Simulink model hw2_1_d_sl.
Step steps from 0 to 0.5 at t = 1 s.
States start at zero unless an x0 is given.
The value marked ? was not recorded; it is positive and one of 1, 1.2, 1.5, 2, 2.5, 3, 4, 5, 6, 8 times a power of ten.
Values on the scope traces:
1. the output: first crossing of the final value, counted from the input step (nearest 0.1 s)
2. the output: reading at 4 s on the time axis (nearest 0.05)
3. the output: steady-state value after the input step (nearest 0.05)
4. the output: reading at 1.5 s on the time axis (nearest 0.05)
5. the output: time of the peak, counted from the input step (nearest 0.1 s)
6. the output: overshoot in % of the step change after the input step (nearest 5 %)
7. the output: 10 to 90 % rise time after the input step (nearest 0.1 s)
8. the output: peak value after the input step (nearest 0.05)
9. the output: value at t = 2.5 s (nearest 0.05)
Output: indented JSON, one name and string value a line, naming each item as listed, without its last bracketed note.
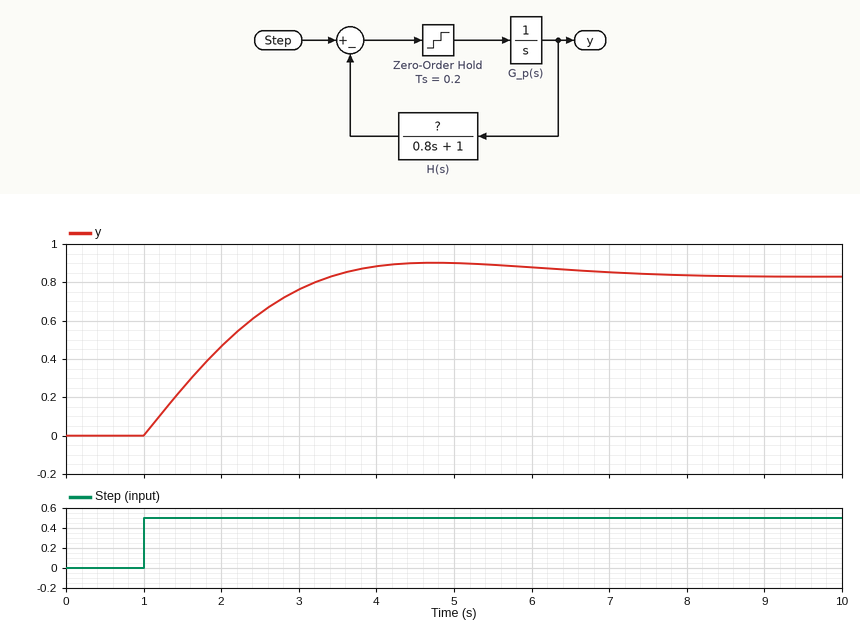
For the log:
{
  "the output: first crossing of the final value, counted from the input step": "2.4 s",
  "the output: reading at 4 s on the time axis": "0.90",
  "the output: steady-state value after the input step": "0.85",
  "the output: reading at 1.5 s on the time axis": "0.25",
  "the output: time of the peak, counted from the input step": "3.8 s",
  "the output: overshoot in % of the step change after the input step": "10 %",
  "the output: 10 to 90 % rise time after the input step": "1.8 s",
  "the output: peak value after the input step": "0.90",
  "the output: value at t = 2.5 s": "0.65"
}
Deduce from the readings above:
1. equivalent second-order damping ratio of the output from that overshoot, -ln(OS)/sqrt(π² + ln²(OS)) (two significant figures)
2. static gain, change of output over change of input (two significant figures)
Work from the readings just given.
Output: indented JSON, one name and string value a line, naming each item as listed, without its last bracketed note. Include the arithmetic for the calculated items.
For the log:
{
  "equivalent second-order damping ratio of the output from that overshoot, -ln(OS)/sqrt(π² + ln²(OS))": "ln(0.1) = -2.303; 2.303 / sqrt(9.870 + 5.302) = 0.59",
  "static gain, change of output over change of input": "(0.85 - 0) / (0.5 - 0) = 1.7"
}
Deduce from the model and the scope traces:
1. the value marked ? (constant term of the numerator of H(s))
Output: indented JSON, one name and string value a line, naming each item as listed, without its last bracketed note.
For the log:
{
  "the value marked ? (constant term of the numerator of H(s))": "0.6"
}
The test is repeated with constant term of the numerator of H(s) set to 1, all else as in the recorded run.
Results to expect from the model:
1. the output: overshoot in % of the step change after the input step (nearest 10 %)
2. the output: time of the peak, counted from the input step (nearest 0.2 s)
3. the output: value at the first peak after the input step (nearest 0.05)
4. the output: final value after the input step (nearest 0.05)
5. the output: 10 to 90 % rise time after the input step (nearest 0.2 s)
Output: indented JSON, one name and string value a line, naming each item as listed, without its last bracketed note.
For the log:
{
  "the output: overshoot in % of the step change after the input step": "30 %",
  "the output: time of the peak, counted from the input step": "2.2 s",
  "the output: value at the first peak after the input step": "0.65",
  "the output: final value after the input step": "0.50",
  "the output: 10 to 90 % rise time after the input step": "1.0 s"
}
